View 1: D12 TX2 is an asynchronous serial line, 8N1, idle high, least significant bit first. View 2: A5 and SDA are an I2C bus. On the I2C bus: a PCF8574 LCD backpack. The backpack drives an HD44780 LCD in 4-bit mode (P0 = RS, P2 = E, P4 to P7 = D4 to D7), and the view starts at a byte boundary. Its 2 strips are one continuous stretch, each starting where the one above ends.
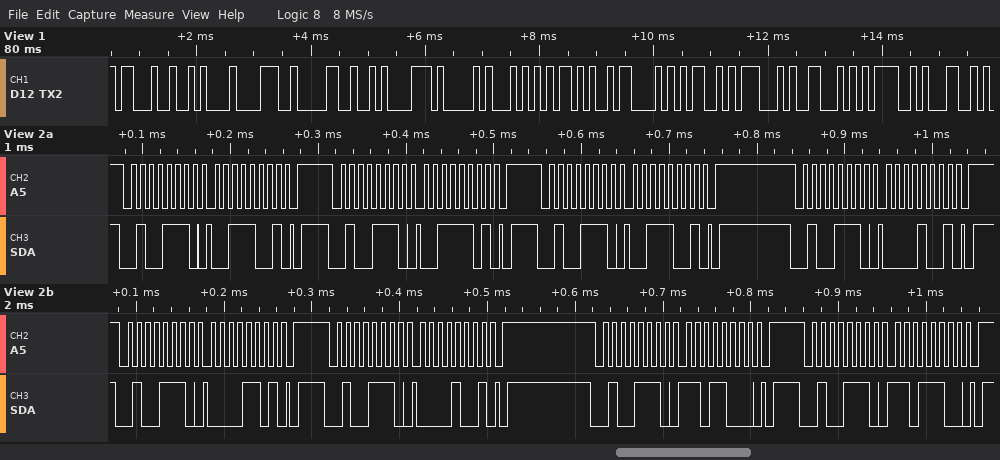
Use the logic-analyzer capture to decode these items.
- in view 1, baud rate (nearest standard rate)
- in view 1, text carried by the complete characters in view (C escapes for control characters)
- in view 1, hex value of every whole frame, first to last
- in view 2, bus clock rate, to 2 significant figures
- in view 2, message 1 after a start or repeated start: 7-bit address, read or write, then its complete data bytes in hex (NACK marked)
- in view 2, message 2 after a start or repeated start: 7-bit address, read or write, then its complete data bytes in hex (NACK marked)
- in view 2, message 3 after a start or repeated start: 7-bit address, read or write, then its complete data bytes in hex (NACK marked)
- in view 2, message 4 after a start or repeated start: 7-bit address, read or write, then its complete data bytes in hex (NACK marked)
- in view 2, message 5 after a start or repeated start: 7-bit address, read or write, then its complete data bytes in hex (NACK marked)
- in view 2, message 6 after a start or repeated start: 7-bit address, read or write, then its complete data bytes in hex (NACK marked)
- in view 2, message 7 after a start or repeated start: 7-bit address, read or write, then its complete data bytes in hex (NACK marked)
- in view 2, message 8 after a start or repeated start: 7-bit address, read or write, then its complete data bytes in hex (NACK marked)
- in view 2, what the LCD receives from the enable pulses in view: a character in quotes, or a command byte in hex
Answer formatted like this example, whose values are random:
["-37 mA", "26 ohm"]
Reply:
["9600 baud", "\"#\\n80\\nAT+CMGF=1\"", "23 0A 38 30 0A 41 54 2B 43 4D 47 46 3D 31", "100 kHz", "0x27 write: 39", "0x27 write: 3D", "0x27 write: 39", "0x27 write: 09", "0x27 write: 0D", "0x27 write: 09", "0x27 write: D8", "0x27 write: DC", "'0'"]
